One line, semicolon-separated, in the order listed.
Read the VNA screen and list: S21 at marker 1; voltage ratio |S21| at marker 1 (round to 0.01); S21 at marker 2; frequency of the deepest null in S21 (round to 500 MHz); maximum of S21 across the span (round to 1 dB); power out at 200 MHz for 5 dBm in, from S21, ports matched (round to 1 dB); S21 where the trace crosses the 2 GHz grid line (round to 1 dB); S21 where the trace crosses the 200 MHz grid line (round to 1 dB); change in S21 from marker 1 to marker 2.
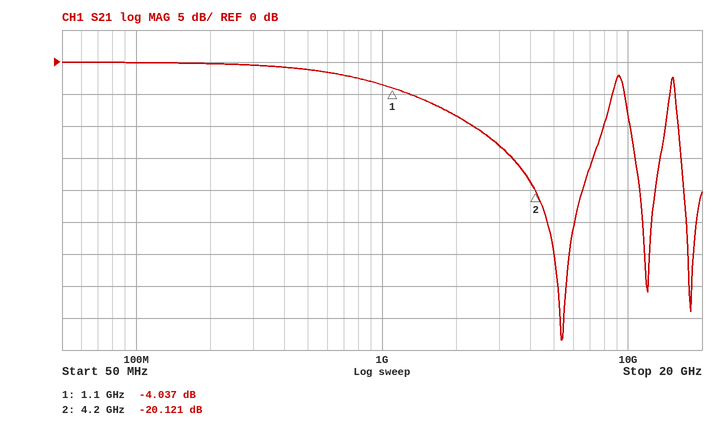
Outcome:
-4.037 dB; 0.63; -20.121 dB; 5.5 GHz; 0 dB; 5 dBm; -8 dB; 0 dB; -16.084 dB
